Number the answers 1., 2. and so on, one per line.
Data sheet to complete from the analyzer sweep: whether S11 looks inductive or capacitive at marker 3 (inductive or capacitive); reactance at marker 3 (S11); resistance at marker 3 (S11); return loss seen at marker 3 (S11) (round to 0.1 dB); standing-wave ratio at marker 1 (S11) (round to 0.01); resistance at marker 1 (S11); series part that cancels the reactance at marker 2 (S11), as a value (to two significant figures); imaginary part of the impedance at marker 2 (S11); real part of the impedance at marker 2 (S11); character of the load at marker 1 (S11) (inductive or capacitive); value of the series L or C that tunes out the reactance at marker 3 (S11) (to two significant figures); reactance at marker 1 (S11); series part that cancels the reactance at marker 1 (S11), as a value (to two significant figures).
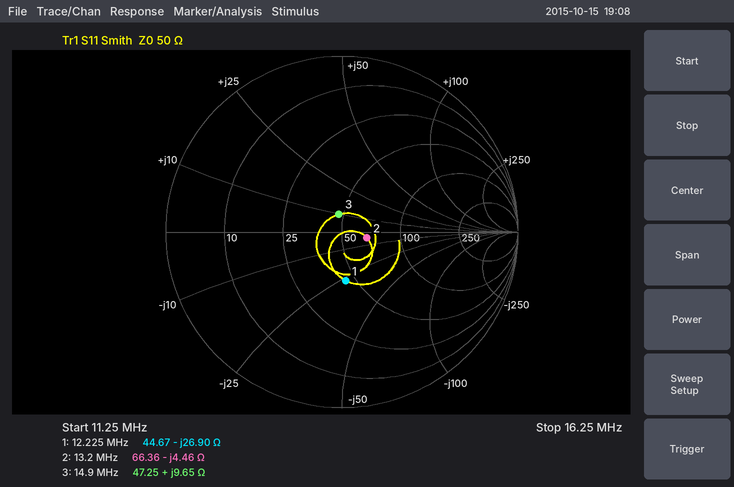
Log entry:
1. inductive
2. +9.65 Ω
3. 47.25 Ω
4. 19.8 dB
5. 1.77
6. 44.67 Ω
7. 54 nH
8. -4.46 Ω
9. 66.36 Ω
10. capacitive
11. 1.1 nF
12. -26.90 Ω
13. 350 nH
